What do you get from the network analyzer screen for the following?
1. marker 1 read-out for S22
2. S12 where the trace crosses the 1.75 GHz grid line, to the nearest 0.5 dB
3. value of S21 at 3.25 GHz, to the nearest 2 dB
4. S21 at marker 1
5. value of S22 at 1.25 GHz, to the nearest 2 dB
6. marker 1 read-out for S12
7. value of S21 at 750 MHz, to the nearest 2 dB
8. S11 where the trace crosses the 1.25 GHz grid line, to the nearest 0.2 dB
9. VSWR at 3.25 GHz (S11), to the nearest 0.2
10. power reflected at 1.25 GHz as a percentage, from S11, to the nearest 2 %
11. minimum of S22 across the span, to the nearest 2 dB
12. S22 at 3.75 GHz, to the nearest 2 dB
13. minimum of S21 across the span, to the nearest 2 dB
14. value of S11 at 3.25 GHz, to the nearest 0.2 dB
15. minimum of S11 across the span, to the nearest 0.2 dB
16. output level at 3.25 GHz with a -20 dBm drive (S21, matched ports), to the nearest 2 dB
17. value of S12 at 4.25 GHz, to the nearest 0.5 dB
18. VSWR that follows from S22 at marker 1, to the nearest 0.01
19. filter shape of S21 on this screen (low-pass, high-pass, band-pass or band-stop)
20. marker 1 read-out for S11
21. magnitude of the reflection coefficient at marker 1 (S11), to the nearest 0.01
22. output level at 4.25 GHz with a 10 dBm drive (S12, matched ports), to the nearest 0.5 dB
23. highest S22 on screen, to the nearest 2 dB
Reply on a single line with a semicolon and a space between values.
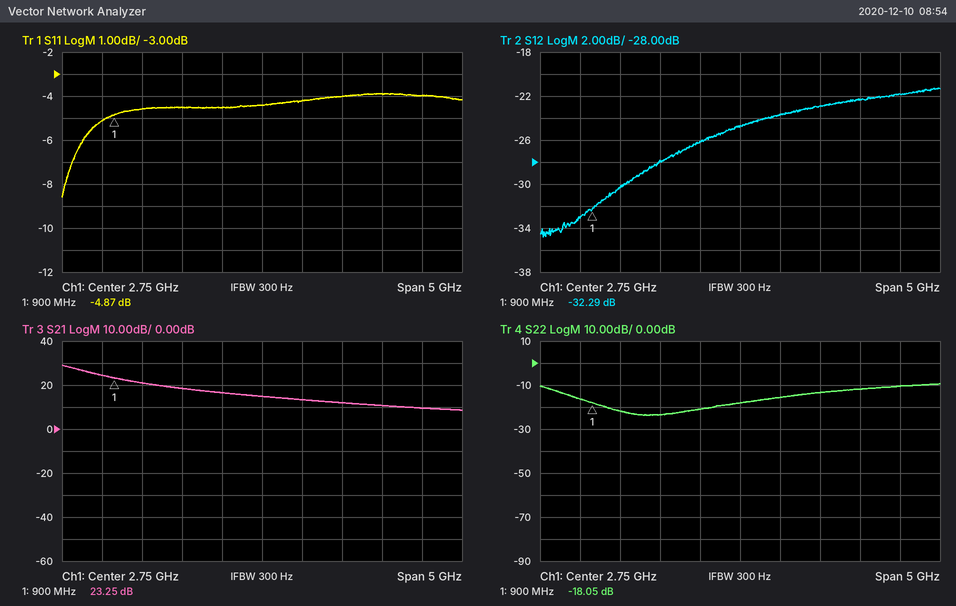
-18.05 dB; -28.0 dB; 14 dB; 23.25 dB; -22 dB; -32.29 dB; 24 dB; -4.6 dB; 4.2; 34 %; -24 dB; -14 dB; 8 dB; -4.2 dB; -8.6 dB; -6 dBm; -22.5 dB; 1.29; low-pass; -4.87 dB; 0.57; -12.5 dBm; -10 dB
